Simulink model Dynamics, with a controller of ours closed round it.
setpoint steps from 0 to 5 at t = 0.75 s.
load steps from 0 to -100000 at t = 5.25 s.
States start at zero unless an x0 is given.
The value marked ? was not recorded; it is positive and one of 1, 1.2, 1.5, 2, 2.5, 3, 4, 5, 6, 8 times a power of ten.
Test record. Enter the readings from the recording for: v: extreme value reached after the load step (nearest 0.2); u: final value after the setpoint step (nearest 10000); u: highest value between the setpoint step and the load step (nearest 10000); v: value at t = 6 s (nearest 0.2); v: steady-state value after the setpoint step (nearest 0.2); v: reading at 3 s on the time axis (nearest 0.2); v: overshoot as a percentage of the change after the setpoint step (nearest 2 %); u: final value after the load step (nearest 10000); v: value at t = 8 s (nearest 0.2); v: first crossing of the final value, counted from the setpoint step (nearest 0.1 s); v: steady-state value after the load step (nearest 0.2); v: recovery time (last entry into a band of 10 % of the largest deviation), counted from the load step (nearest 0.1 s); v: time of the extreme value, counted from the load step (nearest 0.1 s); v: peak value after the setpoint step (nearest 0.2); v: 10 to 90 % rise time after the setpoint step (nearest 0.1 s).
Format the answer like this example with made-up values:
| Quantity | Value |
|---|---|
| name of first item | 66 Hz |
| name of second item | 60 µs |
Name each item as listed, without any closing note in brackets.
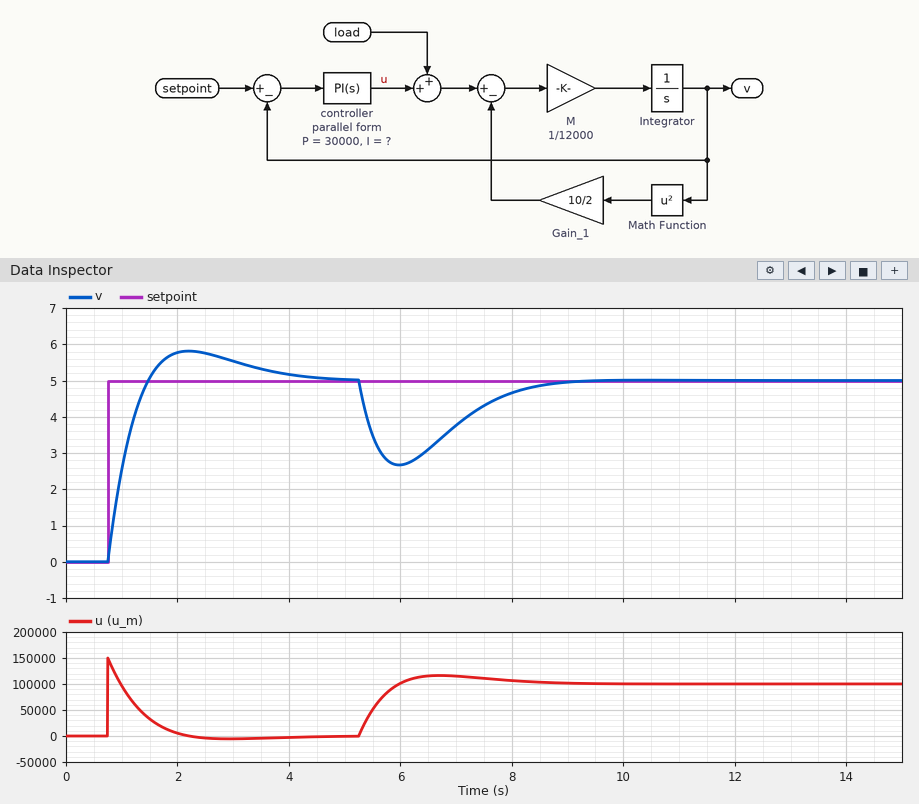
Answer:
| Quantity | Value |
|---|---|
| v: extreme value reached after the load step | 2.6 |
| u: final value after the setpoint step | 0 |
| u: highest value between the setpoint step and the load step | 150000 |
| v: value at t = 6 s | 2.6 |
| v: steady-state value after the setpoint step | 5.0 |
| v: reading at 3 s on the time axis | 5.6 |
| v: overshoot as a percentage of the change after the setpoint step | 16 % |
| u: final value after the load step | 100000 |
| v: value at t = 8 s | 4.6 |
| v: first crossing of the final value, counted from the setpoint step | 0.7 s |
| v: steady-state value after the load step | 5.0 |
| v: recovery time (last entry into a band of 10 % of the largest deviation), counted from the load step | 3.0 s |
| v: time of the extreme value, counted from the load step | 0.7 s |
| v: peak value after the setpoint step | 5.8 |
| v: 10 to 90 % rise time after the setpoint step | 0.5 s |
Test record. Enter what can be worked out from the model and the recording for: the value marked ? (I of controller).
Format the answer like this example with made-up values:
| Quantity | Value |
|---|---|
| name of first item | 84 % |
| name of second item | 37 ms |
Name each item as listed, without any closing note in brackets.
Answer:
| Quantity | Value |
|---|---|
| the value marked ? | 25000 |
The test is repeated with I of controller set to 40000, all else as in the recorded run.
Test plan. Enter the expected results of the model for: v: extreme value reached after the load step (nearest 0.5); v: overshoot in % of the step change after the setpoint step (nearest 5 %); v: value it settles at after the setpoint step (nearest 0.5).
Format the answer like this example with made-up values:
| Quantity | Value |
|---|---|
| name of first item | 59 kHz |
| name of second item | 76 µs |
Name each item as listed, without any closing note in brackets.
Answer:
| Quantity | Value |
|---|---|
| v: extreme value reached after the load step | 3.0 |
| v: overshoot in % of the step change after the setpoint step | 20 % |
| v: value it settles at after the setpoint step | 5.0 |
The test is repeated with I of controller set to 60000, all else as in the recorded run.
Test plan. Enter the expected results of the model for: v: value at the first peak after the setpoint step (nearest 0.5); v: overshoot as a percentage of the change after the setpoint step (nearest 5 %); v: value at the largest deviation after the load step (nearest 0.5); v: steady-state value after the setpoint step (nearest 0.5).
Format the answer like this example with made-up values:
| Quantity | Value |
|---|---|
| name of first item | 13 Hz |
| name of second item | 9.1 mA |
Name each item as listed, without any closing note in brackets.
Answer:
| Quantity | Value |
|---|---|
| v: value at the first peak after the setpoint step | 6.5 |
| v: overshoot as a percentage of the change after the setpoint step | 25 % |
| v: value at the largest deviation after the load step | 3.0 |
| v: steady-state value after the setpoint step | 5.0 |
